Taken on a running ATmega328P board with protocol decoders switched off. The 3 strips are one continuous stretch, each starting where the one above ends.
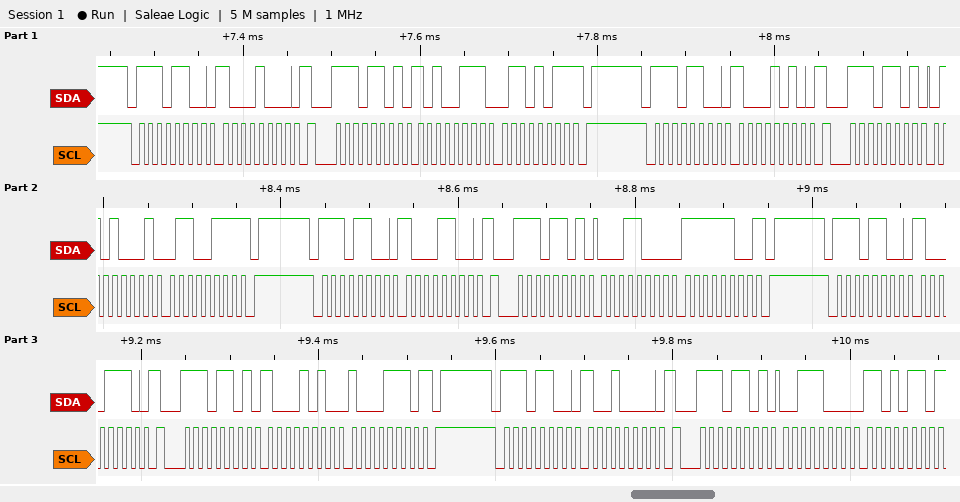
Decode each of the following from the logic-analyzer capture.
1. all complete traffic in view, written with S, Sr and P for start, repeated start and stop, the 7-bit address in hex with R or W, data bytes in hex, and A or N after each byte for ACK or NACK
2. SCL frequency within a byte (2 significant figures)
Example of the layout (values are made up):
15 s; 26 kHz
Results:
S 76W A 88 A Sr 76R A A7 A 6B N P S 76W A 8A A Sr 76R A 51 A 67 N P S 76W A 8C A Sr 76R A 18 A FC N P S 76W A 8E A Sr 76R A 8A A 8E N P S 76W A 90 A Sr 76R A 38 A D6 N; 100 kHz
